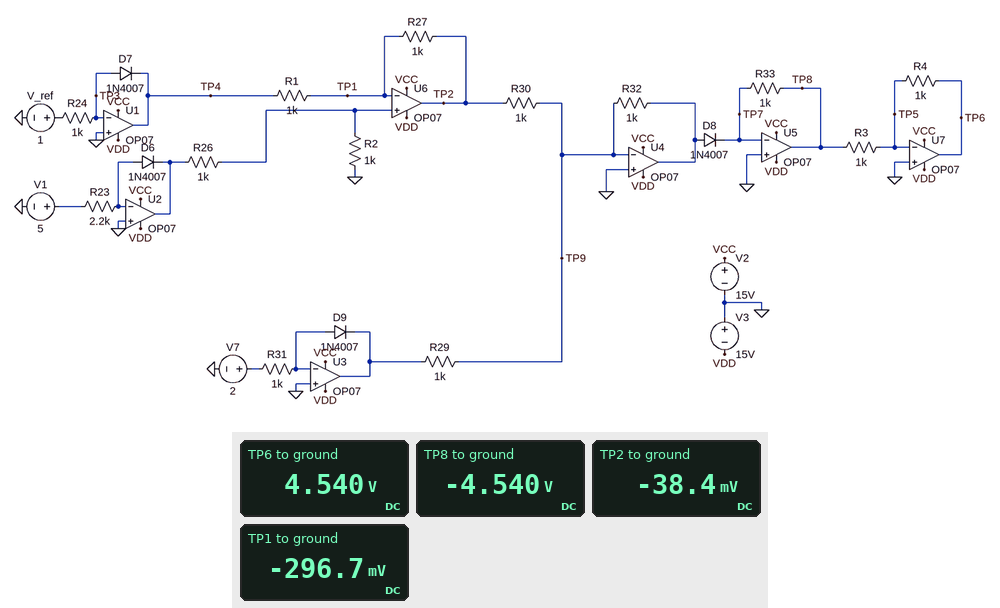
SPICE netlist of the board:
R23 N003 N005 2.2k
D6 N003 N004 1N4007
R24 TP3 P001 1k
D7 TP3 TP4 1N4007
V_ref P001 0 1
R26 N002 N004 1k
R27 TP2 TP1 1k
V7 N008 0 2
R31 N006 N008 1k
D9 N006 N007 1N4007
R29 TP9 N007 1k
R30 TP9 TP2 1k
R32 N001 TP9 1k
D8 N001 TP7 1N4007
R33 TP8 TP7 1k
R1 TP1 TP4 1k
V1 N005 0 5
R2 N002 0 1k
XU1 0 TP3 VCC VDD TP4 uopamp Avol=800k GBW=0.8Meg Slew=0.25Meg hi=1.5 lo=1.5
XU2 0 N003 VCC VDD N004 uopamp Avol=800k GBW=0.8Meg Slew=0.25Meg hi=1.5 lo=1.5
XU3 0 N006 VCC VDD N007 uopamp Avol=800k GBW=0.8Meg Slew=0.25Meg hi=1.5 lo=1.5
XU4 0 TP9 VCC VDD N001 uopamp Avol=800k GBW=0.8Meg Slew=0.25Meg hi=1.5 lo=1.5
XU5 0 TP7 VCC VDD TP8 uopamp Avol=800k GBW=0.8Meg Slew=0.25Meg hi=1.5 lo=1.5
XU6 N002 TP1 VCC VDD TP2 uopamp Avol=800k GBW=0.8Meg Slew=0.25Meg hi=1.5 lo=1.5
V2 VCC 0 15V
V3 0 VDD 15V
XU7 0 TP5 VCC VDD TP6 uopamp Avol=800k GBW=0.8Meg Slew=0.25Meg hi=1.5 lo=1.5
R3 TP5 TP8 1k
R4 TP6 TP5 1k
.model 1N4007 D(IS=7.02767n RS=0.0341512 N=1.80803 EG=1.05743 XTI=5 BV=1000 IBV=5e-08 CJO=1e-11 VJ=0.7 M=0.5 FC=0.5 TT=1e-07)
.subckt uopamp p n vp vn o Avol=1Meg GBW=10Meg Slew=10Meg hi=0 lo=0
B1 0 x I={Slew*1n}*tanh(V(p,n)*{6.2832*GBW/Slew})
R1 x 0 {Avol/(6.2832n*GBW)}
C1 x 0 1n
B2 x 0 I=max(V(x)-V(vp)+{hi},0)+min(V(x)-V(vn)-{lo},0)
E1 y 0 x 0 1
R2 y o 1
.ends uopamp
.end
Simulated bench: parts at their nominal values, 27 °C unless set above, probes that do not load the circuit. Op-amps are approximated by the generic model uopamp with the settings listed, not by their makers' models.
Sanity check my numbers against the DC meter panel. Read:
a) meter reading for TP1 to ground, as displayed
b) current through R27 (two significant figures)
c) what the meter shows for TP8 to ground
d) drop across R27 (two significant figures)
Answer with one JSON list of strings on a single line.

["-296.7 mV", "260 µA", "-4.540 V", "260 mV"]
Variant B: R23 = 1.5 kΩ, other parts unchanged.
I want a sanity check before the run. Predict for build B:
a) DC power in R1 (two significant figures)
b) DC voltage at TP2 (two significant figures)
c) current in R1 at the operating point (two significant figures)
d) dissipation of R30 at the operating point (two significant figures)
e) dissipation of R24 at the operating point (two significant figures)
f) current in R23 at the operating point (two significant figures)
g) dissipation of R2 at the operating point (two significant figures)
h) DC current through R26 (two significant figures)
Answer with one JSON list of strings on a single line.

["62 µW", "-56 mV", "250 µA", "3.2 µW", "1.0 mW", "3.3 mA", "93 µW", "310 µA"]
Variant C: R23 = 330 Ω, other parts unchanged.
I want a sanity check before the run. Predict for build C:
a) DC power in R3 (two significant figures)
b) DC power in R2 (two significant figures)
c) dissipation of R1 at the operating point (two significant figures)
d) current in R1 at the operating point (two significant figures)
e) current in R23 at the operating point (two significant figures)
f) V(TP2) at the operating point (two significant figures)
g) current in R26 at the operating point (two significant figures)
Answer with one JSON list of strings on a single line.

["180 mW", "120 µW", "46 µW", "210 µA", "15 mA", "-130 mV", "340 µA"]
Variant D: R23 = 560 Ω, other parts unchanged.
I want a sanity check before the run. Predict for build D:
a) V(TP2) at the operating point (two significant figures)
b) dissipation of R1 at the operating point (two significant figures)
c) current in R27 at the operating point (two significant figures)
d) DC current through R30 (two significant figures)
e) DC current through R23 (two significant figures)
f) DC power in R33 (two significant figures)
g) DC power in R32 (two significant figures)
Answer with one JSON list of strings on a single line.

["-100 mV", "51 µW", "230 µA", "100 µA", "8.9 mA", "180 mW", "480 µW"]
